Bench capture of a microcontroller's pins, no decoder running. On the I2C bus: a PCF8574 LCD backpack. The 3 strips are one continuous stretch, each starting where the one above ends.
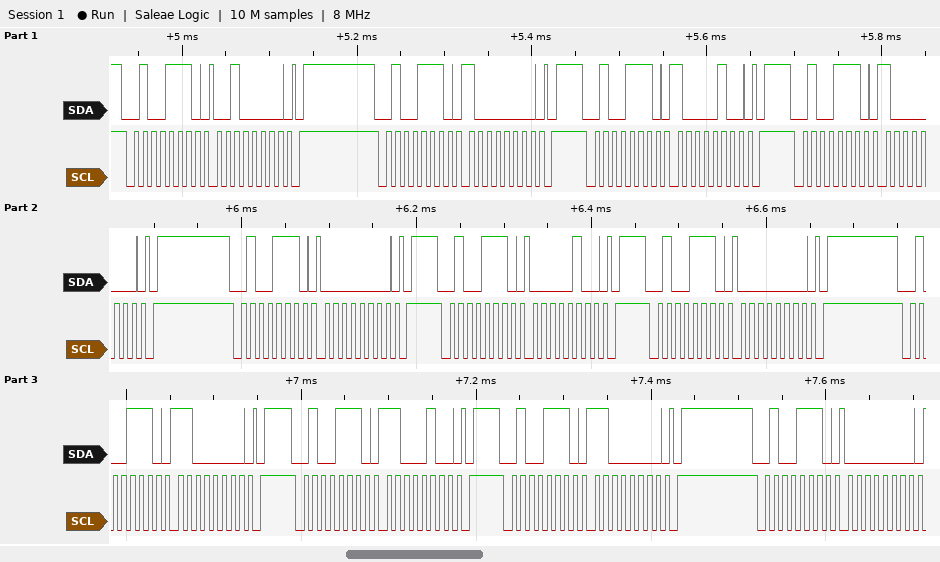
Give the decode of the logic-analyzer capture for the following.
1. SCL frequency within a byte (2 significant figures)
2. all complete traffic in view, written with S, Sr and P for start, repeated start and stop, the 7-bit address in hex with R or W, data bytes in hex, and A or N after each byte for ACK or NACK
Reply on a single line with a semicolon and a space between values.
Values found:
100 kHz; S 27W A 20 A P S 27W A 80 A P S 27W A 84 A P S 27W A 80 A P S 27W A 00 A P S 27W A 04 A P S 27W A 00 A P S 27W A C0 A P S 27W A C4 A P S 27W A C0 A P S 27W A 00 A
